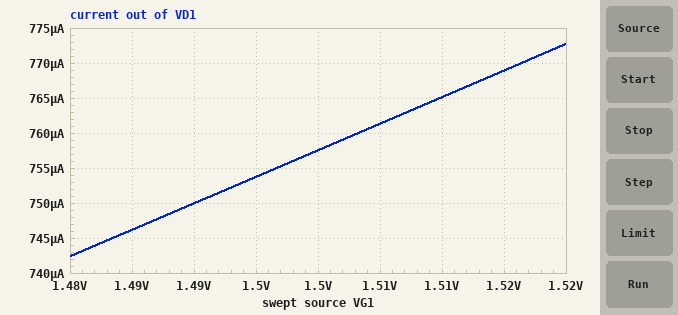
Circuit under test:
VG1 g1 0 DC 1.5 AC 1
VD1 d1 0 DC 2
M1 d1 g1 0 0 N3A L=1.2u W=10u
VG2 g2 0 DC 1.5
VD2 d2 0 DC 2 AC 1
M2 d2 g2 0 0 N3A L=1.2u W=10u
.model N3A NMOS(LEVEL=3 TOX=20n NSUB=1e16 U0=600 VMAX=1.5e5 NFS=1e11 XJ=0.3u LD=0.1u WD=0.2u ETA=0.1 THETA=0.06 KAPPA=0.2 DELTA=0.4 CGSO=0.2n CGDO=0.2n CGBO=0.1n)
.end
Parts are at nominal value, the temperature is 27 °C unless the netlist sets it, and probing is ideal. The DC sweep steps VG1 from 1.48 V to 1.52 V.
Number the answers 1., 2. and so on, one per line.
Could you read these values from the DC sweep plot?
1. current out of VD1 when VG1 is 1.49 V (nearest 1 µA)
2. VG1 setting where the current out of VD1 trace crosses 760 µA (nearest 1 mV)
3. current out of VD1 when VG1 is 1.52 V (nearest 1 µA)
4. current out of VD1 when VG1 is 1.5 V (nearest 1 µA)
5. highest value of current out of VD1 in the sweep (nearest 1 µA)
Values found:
1. 746 µA
2. 1.503 V
3. 769 µA
4. 754 µA
5. 773 µA
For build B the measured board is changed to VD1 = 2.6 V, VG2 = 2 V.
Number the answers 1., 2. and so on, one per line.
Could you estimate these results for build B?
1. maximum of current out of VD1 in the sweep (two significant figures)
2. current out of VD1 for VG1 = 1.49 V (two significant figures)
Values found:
1. 830 µA
2. 800 µA
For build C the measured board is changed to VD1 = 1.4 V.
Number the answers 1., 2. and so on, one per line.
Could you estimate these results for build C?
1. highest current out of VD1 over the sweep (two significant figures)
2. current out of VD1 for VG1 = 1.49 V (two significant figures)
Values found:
1. 720 µA
2. 690 µA
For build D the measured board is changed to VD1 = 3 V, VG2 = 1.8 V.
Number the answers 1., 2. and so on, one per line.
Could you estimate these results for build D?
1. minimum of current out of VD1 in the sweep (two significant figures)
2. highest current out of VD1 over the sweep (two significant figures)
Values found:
1. 830 µA
2. 860 µA
